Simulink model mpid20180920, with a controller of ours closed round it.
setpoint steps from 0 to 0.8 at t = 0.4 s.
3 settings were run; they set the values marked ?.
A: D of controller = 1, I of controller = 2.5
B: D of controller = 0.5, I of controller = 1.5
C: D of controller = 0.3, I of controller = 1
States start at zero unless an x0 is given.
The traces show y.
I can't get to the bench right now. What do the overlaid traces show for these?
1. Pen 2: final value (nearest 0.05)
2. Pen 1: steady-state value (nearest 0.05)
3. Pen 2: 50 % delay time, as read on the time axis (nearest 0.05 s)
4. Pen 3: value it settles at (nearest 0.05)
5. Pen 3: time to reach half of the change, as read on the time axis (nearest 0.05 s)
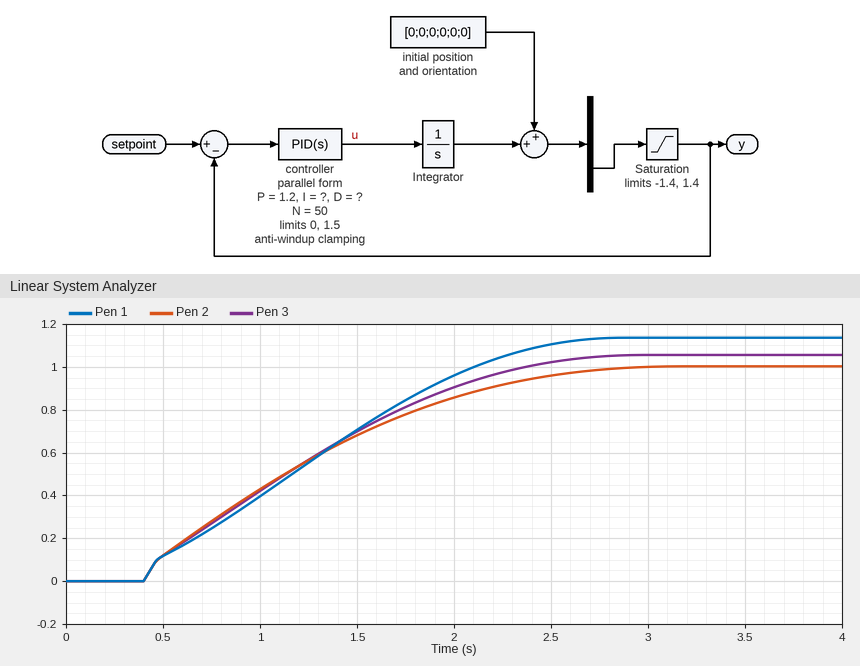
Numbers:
1.00
1.15
1.15 s
1.05
1.20 s
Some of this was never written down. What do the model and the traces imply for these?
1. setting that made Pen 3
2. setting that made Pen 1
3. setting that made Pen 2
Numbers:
B
A
C
